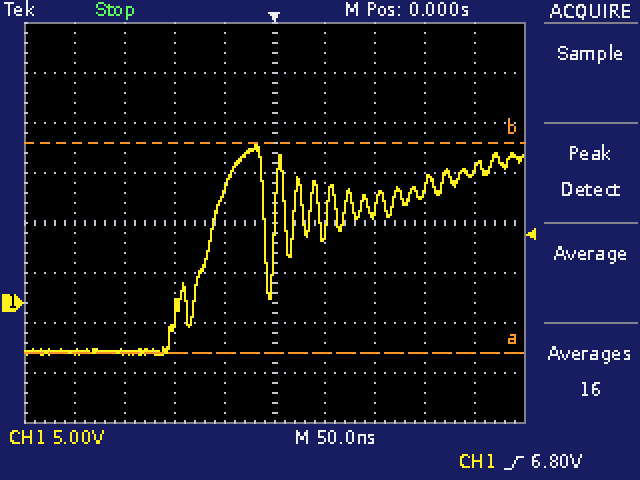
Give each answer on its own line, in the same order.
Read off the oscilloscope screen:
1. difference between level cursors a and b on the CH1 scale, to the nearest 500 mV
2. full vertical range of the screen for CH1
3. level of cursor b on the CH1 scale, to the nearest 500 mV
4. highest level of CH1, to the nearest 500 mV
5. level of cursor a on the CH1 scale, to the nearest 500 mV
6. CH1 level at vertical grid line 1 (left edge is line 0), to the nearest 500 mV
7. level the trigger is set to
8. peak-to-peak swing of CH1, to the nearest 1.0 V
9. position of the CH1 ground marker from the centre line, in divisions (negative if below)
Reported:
21.0 V
40 V
16.0 V
16.0 V
-5.0 V
-5.0 V
6.80 V
21.0 V
-1.6 div
